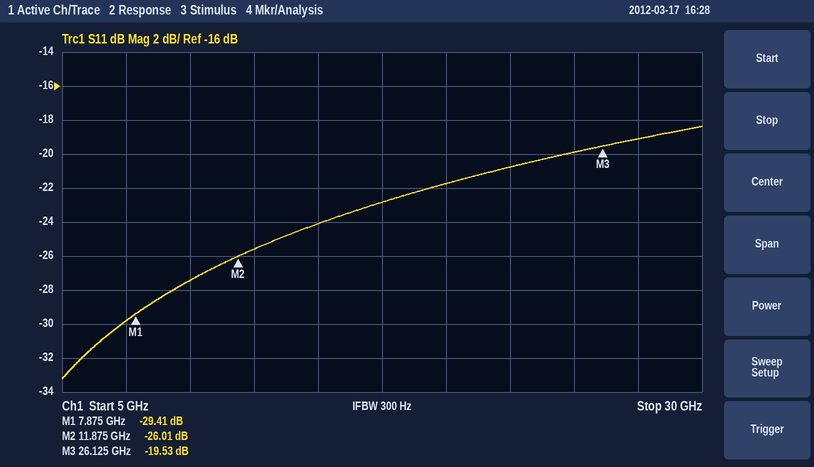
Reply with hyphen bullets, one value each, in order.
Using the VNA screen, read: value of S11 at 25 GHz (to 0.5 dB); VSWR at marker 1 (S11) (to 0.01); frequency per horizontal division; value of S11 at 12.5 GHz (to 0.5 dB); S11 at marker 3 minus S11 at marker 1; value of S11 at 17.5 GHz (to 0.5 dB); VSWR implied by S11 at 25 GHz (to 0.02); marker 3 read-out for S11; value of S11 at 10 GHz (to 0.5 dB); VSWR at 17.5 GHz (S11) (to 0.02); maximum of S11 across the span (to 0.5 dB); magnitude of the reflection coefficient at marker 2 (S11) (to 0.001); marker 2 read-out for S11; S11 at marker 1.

- -20.0 dB
- 1.07
- 2.5 GHz
- -25.5 dB
- 9.88 dB
- -23.0 dB
- 1.22
- -19.53 dB
- -27.5 dB
- 1.16
- -18.5 dB
- 0.050
- -26.01 dB
- -29.41 dB
